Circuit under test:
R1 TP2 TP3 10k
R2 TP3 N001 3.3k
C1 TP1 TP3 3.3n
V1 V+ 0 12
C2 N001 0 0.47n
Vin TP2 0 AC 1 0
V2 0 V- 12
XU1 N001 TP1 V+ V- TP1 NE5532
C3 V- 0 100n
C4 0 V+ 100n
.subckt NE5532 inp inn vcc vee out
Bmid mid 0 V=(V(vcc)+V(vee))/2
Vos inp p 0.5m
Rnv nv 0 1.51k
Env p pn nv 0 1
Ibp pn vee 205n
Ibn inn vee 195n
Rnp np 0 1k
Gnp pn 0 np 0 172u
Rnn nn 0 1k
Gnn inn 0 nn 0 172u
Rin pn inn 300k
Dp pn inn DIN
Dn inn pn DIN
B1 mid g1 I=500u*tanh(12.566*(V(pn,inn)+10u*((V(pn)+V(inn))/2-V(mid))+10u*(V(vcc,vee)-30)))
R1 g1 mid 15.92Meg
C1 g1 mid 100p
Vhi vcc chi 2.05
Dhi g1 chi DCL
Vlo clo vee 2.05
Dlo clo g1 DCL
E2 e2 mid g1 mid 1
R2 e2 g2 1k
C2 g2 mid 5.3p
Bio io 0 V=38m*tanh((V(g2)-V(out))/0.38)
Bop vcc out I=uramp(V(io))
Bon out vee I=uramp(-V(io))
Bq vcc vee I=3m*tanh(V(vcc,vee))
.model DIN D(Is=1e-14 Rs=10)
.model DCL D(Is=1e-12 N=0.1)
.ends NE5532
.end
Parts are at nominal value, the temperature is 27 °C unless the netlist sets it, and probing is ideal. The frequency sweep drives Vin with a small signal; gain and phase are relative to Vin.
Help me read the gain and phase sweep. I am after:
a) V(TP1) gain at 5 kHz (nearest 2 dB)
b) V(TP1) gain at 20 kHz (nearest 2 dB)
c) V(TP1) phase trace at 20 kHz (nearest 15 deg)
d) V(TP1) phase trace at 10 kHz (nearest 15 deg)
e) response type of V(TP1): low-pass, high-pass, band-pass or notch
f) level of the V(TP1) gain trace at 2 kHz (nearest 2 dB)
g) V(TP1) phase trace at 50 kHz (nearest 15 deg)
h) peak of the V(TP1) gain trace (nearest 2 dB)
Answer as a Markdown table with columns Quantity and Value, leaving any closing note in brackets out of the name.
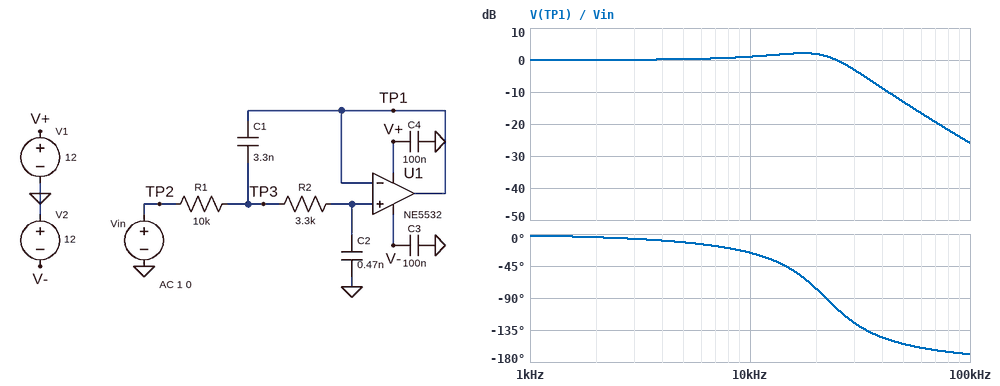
| Quantity | Value |
|---|---|
| V(TP1) gain at 5 kHz | 0 dB |
| V(TP1) gain at 20 kHz | 2 dB |
| V(TP1) phase trace at 20 kHz | -75 deg |
| V(TP1) phase trace at 10 kHz | -30 deg |
| response type of V(TP1): low-pass, high-pass, band-pass or notch | low-pass |
| level of the V(TP1) gain trace at 2 kHz | 0 dB |
| V(TP1) phase trace at 50 kHz | -150 deg |
| peak of the V(TP1) gain trace | 2 dB |
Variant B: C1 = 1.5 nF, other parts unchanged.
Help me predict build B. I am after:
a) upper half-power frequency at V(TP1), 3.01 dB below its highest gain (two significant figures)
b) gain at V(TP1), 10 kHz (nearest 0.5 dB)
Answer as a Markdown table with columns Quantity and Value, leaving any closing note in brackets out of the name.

| Quantity | Value |
|---|---|
| upper half-power frequency at V(TP1), 3.01 dB below its highest gain | 35 kHz |
| gain at V(TP1), 10 kHz | 0 dB |
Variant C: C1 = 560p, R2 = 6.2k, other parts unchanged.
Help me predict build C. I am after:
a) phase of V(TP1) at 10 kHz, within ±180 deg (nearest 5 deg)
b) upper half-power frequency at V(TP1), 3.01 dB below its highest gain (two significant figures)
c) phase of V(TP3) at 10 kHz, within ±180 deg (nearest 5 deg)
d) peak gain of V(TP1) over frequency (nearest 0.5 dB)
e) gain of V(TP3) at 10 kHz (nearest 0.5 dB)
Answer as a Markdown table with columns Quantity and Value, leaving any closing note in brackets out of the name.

| Quantity | Value |
|---|---|
| phase of V(TP1) at 10 kHz, within ±180 deg | -25 deg |
| upper half-power frequency at V(TP1), 3.01 dB below its highest gain | 28 kHz |
| phase of V(TP3) at 10 kHz, within ±180 deg | -15 deg |
| peak gain of V(TP1) over frequency | 0 dB |
| gain of V(TP3) at 10 kHz | -0.5 dB |
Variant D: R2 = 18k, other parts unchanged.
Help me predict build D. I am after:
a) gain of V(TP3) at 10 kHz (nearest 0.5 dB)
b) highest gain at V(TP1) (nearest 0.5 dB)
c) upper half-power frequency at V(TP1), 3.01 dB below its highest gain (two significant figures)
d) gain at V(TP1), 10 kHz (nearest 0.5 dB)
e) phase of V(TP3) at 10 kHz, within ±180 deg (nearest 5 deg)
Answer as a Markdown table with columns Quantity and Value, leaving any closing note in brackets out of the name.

| Quantity | Value |
|---|---|
| gain of V(TP3) at 10 kHz | 2.5 dB |
| highest gain at V(TP1) | 3.0 dB |
| upper half-power frequency at V(TP1), 3.01 dB below its highest gain | 11 kHz |
| gain at V(TP1), 10 kHz | 1.5 dB |
| phase of V(TP3) at 10 kHz, within ±180 deg | -70 deg |
